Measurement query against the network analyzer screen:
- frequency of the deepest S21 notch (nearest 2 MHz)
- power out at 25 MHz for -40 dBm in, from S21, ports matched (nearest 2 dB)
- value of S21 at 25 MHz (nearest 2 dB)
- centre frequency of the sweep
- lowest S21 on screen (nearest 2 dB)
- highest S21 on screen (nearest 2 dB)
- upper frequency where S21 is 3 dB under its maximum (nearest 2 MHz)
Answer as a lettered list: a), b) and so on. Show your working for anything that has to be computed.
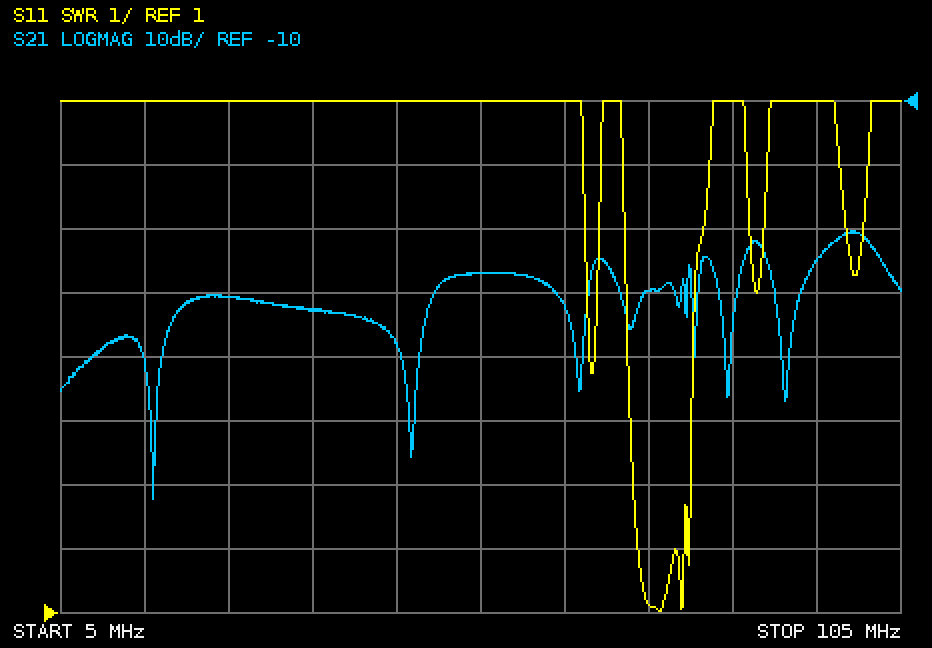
a) 16 MHz
b) -40 dBm + (-40 dB) = -80 dBm
c) -40 dB
d) 55 MHz
e) -72 dB
f) -30 dB
g) 102 MHz
